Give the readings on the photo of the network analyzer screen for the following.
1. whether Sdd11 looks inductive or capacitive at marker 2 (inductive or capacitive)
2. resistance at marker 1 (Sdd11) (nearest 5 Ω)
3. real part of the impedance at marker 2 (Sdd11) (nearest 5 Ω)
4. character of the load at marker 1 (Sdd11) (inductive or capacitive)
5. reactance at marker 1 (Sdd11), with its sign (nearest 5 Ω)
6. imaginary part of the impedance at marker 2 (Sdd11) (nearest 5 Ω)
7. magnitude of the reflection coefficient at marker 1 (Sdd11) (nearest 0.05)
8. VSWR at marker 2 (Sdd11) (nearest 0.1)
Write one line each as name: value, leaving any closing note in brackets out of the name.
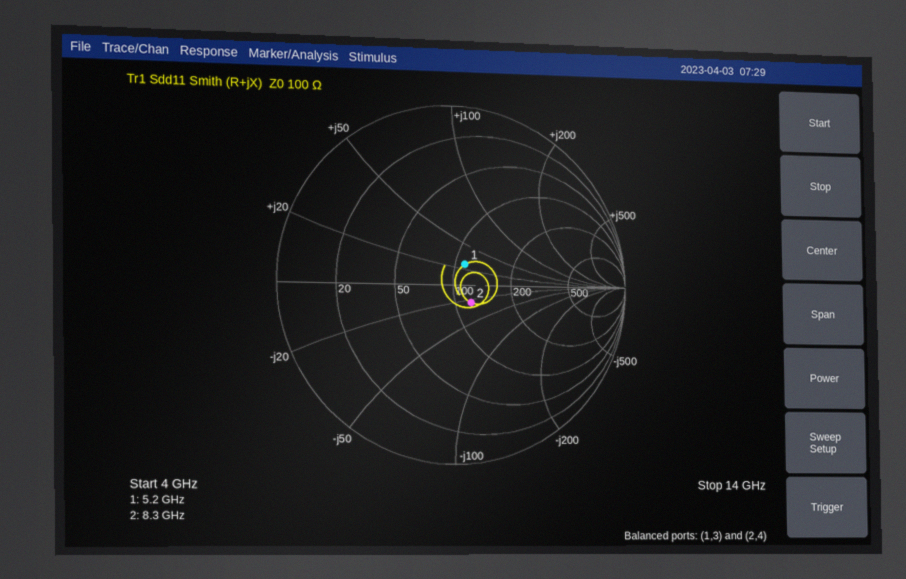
whether Sdd11 looks inductive or capacitive at marker 2: capacitive
resistance at marker 1 (Sdd11): 110 Ω
real part of the impedance at marker 2 (Sdd11): 120 Ω
character of the load at marker 1 (Sdd11): inductive
reactance at marker 1 (Sdd11), with its sign: +25 Ω
imaginary part of the impedance at marker 2 (Sdd11): -25 Ω
magnitude of the reflection coefficient at marker 1 (Sdd11): 0.15
VSWR at marker 2 (Sdd11): 1.3
